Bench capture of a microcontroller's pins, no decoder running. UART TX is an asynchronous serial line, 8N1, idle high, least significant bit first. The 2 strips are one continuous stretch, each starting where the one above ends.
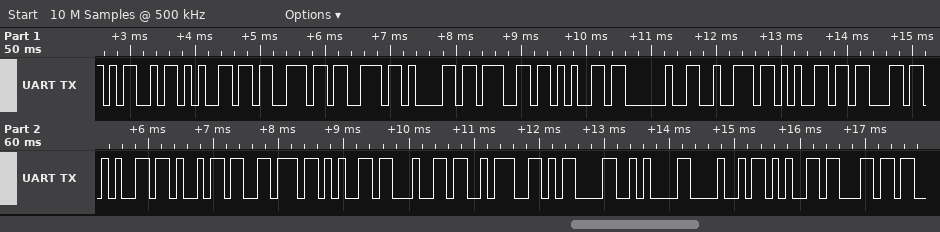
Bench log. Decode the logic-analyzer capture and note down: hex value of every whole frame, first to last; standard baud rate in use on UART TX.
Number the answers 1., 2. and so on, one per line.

1. 0x4D 0x65 0x73 0x73 0x61 0x67 0x65 0x20 0x72 0x65 0x63 0x65 0x69 0x76 0x65 0x64 0x3A 0x0D 0x0A 0x48 0x65 0x6C
2. 9600 baud
